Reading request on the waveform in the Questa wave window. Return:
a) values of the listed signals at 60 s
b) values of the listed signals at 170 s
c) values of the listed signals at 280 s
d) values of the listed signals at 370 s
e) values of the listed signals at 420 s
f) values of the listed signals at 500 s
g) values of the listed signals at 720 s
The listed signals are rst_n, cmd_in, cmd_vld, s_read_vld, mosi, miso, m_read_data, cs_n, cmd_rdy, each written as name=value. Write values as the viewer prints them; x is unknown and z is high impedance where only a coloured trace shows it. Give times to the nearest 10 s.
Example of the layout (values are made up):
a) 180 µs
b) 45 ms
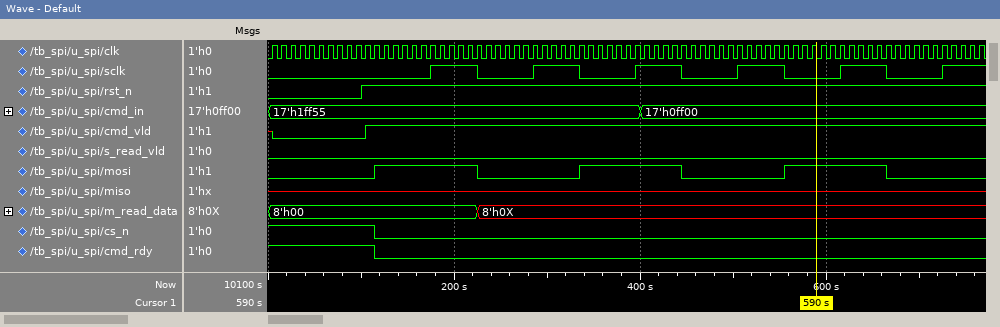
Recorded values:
a) rst_n=0, cmd_in=17'h1ff55, cmd_vld=0, s_read_vld=0, mosi=0, miso=x, m_read_data=8'h00, cs_n=1, cmd_rdy=1
b) rst_n=1, cmd_in=17'h1ff55, cmd_vld=1, s_read_vld=0, mosi=1, miso=x, m_read_data=8'h00, cs_n=0, cmd_rdy=0
c) rst_n=1, cmd_in=17'h1ff55, cmd_vld=1, s_read_vld=0, mosi=0, miso=x, m_read_data=8'h0X, cs_n=0, cmd_rdy=0
d) rst_n=1, cmd_in=17'h1ff55, cmd_vld=1, s_read_vld=0, mosi=1, miso=x, m_read_data=8'h0X, cs_n=0, cmd_rdy=0
e) rst_n=1, cmd_in=17'h0ff00, cmd_vld=1, s_read_vld=0, mosi=1, miso=x, m_read_data=8'h0X, cs_n=0, cmd_rdy=0
f) rst_n=1, cmd_in=17'h0ff00, cmd_vld=1, s_read_vld=0, mosi=0, miso=x, m_read_data=8'h0X, cs_n=0, cmd_rdy=0
g) rst_n=1, cmd_in=17'h0ff00, cmd_vld=1, s_read_vld=0, mosi=0, miso=x, m_read_data=8'h0X, cs_n=0, cmd_rdy=0
